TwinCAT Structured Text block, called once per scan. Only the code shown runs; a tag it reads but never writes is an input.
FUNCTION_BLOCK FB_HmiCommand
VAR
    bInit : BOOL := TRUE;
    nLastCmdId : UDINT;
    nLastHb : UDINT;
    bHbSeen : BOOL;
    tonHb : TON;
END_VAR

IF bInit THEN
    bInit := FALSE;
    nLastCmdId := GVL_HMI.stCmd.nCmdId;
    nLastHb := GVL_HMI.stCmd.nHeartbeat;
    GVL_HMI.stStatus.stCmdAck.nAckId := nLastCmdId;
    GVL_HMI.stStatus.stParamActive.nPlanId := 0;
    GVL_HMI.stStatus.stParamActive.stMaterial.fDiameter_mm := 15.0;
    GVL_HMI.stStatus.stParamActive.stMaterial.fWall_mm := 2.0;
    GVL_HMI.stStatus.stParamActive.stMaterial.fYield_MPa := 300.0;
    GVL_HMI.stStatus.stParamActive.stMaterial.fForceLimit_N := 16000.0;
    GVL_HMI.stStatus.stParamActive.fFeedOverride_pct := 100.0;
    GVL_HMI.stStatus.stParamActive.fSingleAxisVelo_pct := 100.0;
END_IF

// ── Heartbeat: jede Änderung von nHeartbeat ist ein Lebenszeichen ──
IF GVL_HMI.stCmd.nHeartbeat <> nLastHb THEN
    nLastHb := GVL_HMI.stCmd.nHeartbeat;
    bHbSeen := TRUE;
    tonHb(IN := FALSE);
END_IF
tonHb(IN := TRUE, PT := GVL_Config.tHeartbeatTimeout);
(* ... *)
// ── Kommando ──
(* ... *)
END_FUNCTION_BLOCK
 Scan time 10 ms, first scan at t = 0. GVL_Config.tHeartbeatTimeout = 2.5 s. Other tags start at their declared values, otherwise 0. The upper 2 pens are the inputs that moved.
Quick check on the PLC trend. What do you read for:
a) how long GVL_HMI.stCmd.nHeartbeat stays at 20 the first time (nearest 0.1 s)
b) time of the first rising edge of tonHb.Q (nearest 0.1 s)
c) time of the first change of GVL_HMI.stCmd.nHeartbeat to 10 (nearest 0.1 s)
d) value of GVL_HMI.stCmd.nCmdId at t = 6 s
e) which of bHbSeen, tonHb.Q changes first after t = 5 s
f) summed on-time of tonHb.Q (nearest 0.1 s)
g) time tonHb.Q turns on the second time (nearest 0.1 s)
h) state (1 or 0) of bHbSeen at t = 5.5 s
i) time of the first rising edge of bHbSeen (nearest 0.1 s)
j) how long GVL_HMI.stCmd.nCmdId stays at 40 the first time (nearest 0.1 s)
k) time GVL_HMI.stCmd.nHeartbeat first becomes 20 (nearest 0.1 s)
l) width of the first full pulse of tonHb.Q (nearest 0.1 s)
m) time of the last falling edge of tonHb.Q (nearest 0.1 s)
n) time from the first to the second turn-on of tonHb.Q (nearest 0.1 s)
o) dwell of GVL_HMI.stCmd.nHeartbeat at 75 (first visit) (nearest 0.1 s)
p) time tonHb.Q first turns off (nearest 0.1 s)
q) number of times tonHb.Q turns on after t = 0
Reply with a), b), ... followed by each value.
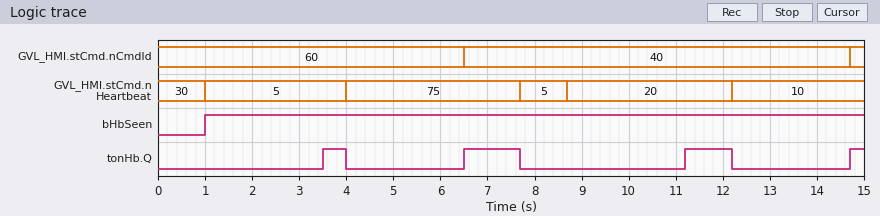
a) 3.5 s
b) 3.5 s
c) 12.2 s
d) 60
e) tonHb.Q
f) 3.0 s
g) 6.5 s
h) 1
i) 1.0 s
j) 8.2 s
k) 8.7 s
l) 0.5 s
m) 12.2 s
n) 3.0 s
o) 3.7 s
p) 4.0 s
q) 4
